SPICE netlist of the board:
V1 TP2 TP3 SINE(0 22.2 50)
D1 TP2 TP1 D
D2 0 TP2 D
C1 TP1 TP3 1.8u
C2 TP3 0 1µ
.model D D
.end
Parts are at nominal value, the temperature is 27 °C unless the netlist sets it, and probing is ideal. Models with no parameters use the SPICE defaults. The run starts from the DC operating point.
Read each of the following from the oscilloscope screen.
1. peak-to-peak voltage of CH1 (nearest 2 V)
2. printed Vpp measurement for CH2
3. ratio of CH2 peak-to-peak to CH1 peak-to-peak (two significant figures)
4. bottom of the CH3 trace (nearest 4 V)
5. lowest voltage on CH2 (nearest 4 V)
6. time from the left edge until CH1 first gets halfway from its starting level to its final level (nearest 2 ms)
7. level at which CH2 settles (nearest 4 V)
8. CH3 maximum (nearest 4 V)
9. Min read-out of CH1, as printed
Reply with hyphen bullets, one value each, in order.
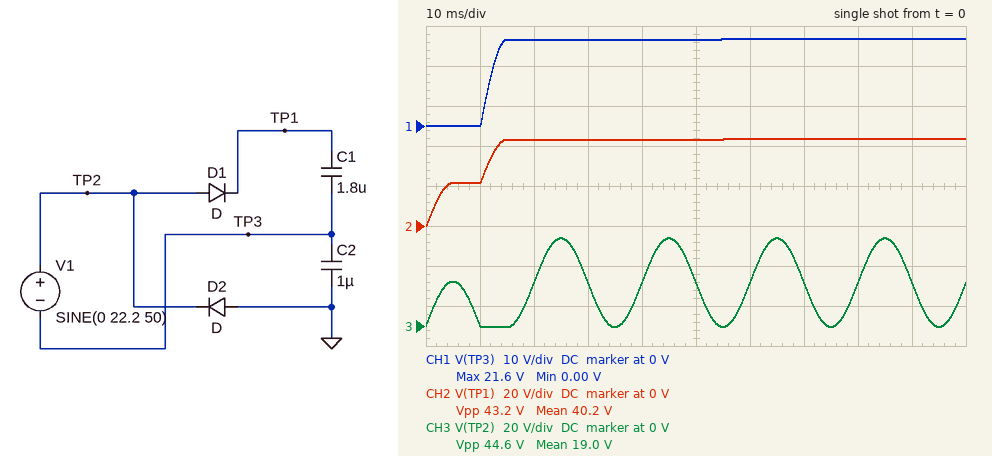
- 22 V
- 43.2 V
- 2.0
- 0 V
- 0 V
- 12 ms
- 44 V
- 44 V
- 0.00 V
